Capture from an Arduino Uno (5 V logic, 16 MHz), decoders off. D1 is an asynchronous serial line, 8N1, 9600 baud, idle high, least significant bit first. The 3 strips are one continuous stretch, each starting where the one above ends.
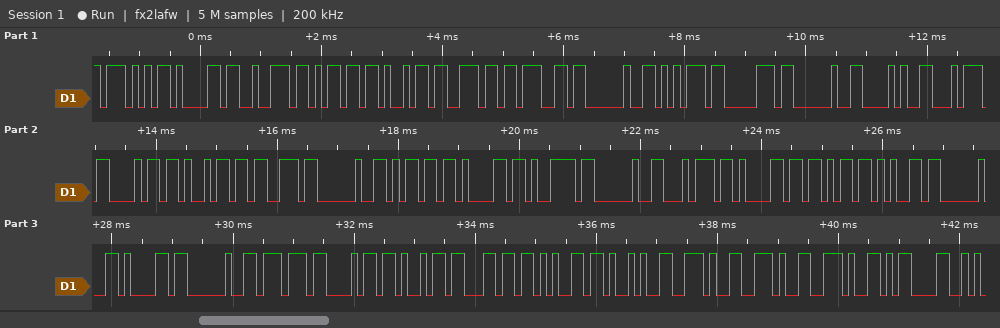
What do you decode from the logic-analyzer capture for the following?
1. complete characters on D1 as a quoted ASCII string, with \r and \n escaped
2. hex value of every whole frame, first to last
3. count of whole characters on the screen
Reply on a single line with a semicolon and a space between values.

"Warming up (this may take a while)...\r"; 0x57 0x61 0x72 0x6D 0x69 0x6E 0x67 0x20 0x75 0x70 0x20 0x28 0x74 0x68 0x69 0x73 0x20 0x6D 0x61 0x79 0x20 0x74 0x61 0x6B 0x65 0x20 0x61 0x20 0x77 0x68 0x69 0x6C 0x65 0x29 0x2E 0x2E 0x2E 0x0D; 38
